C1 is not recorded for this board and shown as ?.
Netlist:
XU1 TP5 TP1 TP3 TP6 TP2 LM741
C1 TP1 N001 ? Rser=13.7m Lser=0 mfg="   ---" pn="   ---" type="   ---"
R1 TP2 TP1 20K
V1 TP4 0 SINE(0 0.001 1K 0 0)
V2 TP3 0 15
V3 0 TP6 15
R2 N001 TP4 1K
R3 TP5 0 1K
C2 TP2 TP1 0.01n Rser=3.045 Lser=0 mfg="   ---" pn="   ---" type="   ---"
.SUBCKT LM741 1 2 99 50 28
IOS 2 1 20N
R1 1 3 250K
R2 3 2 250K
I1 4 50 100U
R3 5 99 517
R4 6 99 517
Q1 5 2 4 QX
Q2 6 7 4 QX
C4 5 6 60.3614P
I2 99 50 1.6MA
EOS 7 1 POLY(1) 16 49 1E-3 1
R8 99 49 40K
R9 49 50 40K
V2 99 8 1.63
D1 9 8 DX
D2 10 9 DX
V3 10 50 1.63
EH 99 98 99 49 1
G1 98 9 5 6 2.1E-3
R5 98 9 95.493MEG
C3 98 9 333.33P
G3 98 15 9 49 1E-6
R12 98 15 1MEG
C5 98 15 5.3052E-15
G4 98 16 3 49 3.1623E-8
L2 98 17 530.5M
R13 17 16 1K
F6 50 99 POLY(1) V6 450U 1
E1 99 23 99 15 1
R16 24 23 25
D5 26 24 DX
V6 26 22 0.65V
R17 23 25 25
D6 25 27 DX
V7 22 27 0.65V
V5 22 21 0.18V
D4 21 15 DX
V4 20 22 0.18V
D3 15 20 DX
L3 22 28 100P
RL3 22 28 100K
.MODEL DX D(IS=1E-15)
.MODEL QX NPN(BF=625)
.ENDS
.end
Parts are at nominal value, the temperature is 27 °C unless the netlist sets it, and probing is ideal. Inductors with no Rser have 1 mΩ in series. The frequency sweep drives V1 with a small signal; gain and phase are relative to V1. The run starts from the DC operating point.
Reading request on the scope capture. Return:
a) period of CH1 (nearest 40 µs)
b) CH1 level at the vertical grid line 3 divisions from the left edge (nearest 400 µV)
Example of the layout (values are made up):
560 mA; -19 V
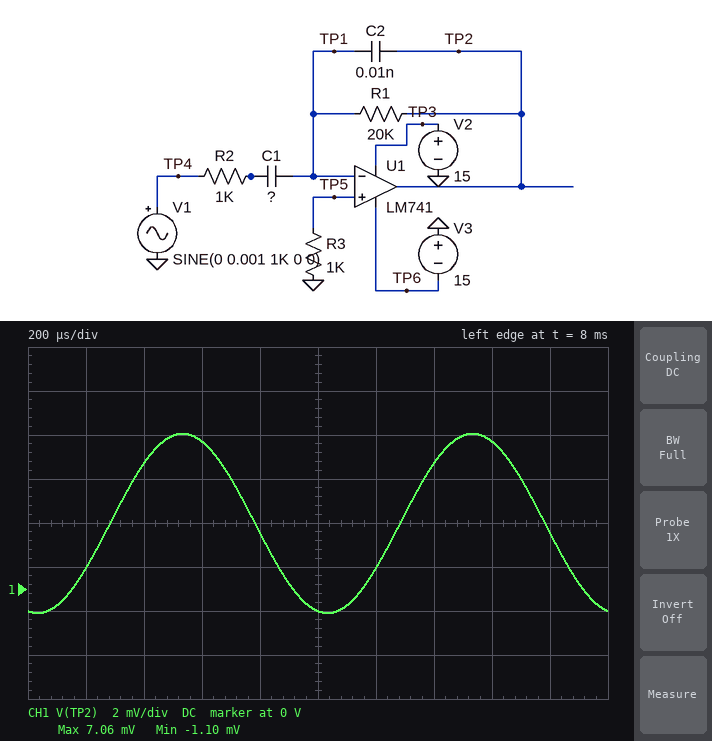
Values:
1.00 ms; 6.8 mV
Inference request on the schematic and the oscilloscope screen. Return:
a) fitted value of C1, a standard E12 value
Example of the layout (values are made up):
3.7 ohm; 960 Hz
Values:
33 nF
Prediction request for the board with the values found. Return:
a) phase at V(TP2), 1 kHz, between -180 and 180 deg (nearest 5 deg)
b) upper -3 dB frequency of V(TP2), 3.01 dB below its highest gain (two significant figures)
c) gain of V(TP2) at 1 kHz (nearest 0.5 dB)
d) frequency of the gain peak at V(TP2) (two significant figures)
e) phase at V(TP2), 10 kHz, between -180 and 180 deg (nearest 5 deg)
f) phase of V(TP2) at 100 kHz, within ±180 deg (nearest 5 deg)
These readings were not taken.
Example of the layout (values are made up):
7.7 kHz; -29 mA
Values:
-100 deg; 50 kHz; 12.0 dB; 15 kHz; -165 deg; 110 deg
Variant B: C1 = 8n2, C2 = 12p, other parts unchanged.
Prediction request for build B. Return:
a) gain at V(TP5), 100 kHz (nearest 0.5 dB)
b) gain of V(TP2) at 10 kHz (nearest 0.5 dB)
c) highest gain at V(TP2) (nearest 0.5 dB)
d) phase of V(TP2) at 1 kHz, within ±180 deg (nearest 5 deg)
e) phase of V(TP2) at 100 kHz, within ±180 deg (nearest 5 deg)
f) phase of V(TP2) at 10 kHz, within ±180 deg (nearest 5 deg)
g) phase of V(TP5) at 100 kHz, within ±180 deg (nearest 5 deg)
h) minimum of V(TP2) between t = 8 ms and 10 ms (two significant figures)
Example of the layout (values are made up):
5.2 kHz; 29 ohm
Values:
-50.0 dB; 20.0 dB; 25.5 dB; -95 deg; 115 deg; -120 deg; 25 deg; 1.9 mV
